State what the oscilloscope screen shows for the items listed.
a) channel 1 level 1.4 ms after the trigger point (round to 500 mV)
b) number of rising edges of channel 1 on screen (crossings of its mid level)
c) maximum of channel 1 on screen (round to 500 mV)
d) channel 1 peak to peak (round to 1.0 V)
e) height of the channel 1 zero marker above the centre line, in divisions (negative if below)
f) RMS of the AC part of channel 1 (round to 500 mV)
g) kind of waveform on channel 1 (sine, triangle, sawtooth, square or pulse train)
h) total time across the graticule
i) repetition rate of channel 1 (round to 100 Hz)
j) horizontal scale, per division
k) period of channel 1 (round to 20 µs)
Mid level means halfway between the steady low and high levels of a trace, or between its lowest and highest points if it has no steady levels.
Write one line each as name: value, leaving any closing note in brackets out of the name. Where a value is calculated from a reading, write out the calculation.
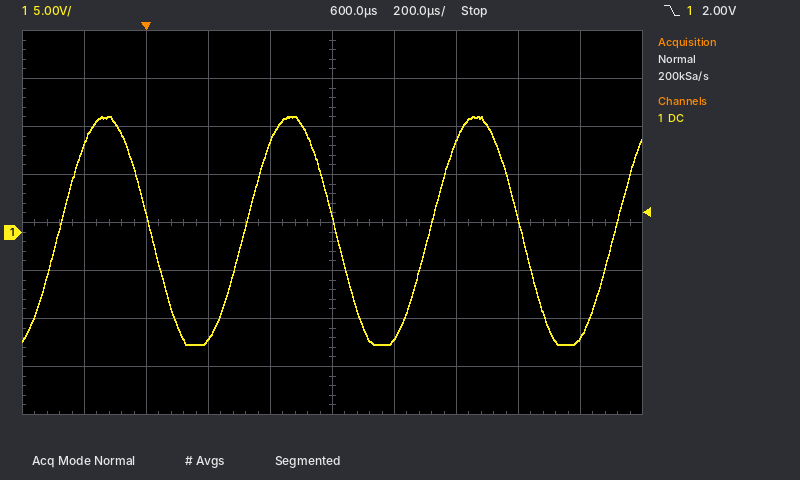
channel 1 level 1.4 ms after the trigger point: -11.0 V
number of rising edges of channel 1 on screen: 4
maximum of channel 1 on screen: 12.0 V
channel 1 peak to peak: 24.0 V
height of the channel 1 zero marker above the centre line, in divisions: -0.2 div
RMS of the AC part of channel 1: 24.0 V / (2√2) ≈ 8.5 V
kind of waveform on channel 1: sine
total time across the graticule: 2 ms
repetition rate of channel 1: 1 / 600 µs ≈ 1.7 kHz
horizontal scale, per division: 200 µs
period of channel 1: 600 µs
